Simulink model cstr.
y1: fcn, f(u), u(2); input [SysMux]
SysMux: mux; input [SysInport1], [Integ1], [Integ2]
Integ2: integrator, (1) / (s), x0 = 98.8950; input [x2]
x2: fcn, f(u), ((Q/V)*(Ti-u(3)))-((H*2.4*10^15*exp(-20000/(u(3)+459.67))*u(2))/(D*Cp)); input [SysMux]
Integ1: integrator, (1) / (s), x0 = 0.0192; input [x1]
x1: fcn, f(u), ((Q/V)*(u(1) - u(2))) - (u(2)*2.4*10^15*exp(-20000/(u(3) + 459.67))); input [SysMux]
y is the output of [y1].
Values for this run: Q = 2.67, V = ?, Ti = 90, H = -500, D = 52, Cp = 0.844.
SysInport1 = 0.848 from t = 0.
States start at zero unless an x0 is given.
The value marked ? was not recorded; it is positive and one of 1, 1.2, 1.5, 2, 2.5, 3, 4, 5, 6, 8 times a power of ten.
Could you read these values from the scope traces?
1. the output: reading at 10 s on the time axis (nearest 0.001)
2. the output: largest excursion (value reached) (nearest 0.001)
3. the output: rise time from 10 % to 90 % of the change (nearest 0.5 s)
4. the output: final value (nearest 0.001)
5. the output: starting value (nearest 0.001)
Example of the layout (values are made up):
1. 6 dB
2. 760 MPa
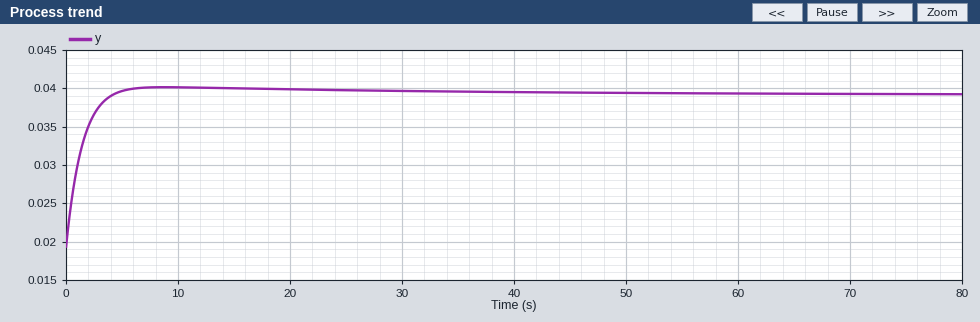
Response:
1. 0.040
2. 0.040
3. 2.5 s
4. 0.039
5. 0.019
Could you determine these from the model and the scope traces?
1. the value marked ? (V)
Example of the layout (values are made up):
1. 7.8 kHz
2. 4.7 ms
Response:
1. 80
